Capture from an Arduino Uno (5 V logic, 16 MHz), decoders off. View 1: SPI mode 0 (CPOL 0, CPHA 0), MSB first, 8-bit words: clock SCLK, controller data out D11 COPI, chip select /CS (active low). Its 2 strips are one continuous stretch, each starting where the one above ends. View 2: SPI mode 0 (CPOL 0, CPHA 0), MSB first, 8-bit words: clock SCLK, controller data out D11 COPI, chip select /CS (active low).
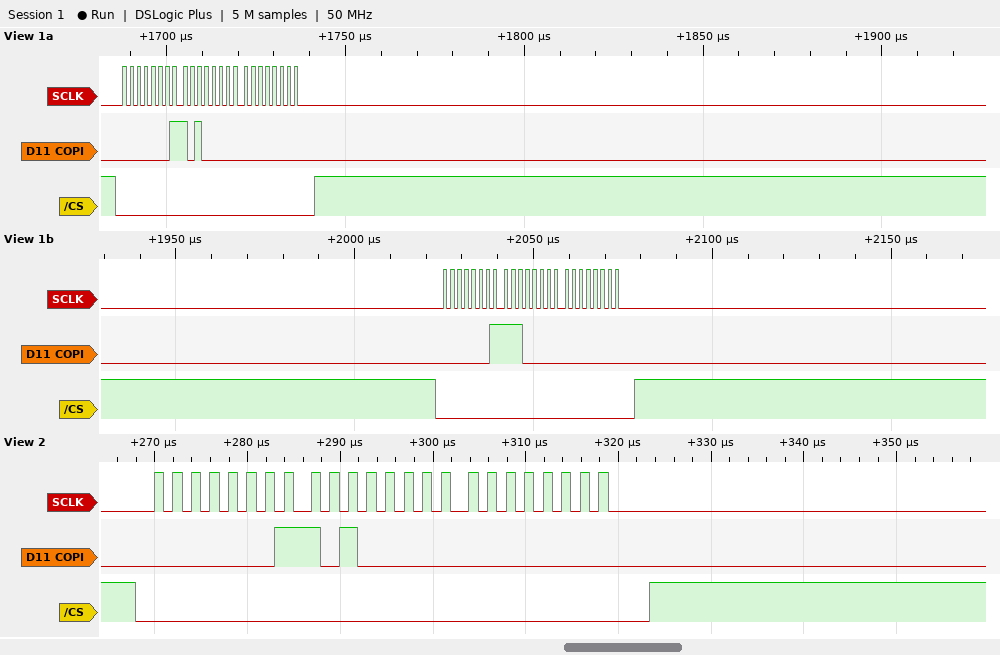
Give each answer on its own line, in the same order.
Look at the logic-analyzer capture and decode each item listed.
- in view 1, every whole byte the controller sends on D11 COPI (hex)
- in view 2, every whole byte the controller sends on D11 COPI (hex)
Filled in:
0x01 0xA0 0x00 0x01 0xE0 0x00
01 A0 00
